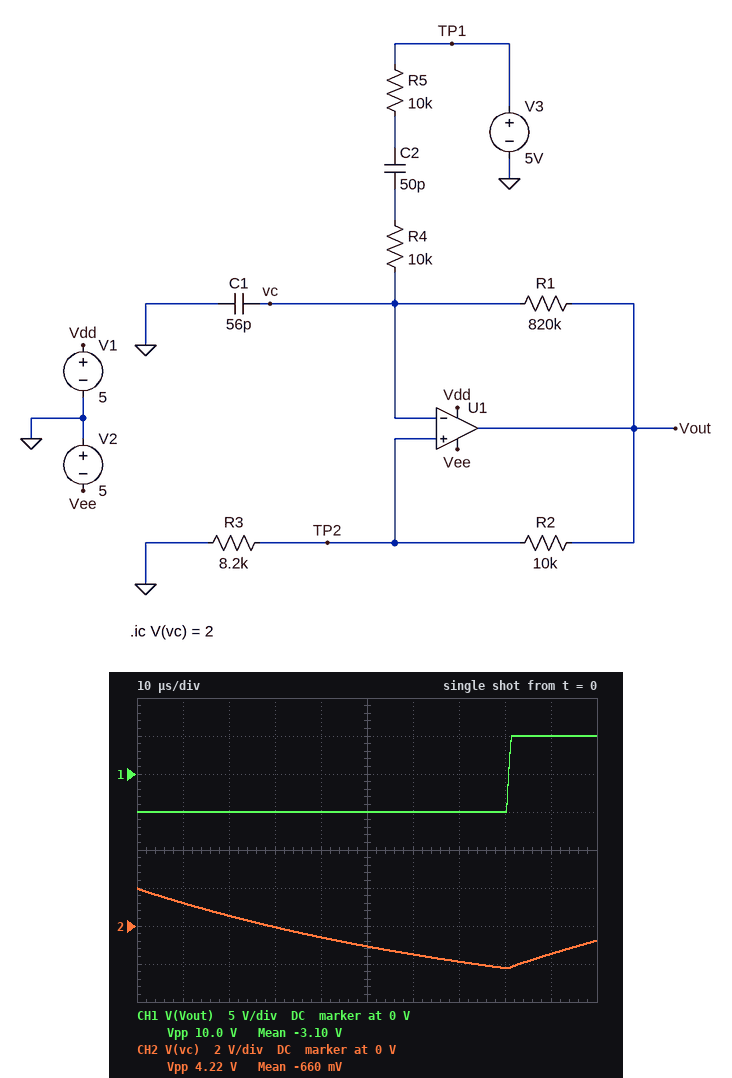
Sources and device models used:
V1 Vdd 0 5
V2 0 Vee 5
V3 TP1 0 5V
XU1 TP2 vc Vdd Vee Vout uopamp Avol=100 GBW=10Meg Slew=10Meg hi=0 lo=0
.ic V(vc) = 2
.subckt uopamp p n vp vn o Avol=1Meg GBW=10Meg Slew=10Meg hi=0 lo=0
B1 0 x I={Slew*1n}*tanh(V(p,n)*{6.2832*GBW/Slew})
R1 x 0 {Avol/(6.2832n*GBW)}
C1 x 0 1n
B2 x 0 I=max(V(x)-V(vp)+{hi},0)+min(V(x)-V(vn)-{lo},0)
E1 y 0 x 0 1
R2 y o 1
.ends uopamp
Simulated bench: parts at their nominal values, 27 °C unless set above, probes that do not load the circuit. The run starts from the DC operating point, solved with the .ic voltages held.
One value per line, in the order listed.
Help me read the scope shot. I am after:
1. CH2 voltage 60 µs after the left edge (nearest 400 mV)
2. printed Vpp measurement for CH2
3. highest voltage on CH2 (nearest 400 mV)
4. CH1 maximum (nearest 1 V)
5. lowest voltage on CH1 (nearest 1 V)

-1.6 V
4.22 V
2.0 V
5 V
-5 V
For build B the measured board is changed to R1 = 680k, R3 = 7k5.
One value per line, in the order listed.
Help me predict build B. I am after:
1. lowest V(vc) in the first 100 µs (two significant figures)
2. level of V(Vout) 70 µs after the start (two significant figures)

-2.1 V
5.0 V
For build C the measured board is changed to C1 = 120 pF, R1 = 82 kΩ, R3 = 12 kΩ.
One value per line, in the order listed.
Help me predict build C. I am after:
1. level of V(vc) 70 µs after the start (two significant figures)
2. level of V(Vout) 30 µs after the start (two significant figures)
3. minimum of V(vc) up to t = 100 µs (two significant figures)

1.4 V
5.0 V
-2.7 V
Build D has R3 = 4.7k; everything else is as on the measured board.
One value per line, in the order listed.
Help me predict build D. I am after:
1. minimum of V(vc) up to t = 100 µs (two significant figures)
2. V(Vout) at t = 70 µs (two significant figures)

-1.6 V
5.0 V
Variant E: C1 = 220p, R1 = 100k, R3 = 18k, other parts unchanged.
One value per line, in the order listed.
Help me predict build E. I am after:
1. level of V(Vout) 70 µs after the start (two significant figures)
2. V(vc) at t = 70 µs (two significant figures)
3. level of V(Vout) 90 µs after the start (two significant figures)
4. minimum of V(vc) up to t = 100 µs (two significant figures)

5.0 V
2.6 V
-5.0 V
-3.2 V
